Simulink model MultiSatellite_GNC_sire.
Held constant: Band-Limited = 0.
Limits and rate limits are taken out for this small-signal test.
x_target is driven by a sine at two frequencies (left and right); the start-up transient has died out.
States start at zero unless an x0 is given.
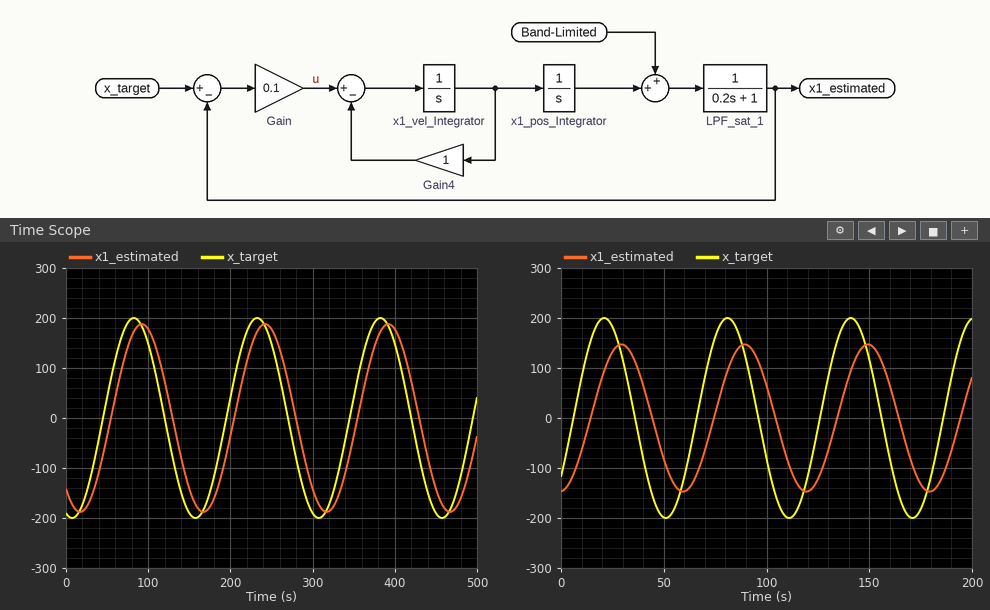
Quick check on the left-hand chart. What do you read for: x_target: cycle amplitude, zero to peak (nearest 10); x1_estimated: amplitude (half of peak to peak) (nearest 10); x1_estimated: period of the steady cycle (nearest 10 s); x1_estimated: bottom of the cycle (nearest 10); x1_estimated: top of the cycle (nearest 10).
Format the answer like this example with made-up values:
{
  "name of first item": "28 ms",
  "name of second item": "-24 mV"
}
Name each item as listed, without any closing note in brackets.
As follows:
{
  "x_target: cycle amplitude, zero to peak": "200",
  "x1_estimated: amplitude (half of peak to peak)": "190",
  "x1_estimated: period of the steady cycle": "150 s",
  "x1_estimated: bottom of the cycle": "-190",
  "x1_estimated: top of the cycle": "190"
}
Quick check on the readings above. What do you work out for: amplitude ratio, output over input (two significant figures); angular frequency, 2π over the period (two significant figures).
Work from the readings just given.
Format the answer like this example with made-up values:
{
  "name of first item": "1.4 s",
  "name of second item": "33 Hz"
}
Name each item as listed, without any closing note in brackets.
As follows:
{
  "amplitude ratio, output over input": "0.95",
  "angular frequency, 2π over the period": "0.042 rad/s"
}
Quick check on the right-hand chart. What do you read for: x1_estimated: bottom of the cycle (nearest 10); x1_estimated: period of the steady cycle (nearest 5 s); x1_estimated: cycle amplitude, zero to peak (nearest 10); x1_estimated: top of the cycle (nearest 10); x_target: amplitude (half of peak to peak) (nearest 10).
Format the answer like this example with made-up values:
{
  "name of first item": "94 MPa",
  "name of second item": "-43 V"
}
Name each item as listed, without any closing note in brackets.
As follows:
{
  "x1_estimated: bottom of the cycle": "-150",
  "x1_estimated: period of the steady cycle": "60 s",
  "x1_estimated: cycle amplitude, zero to peak": "150",
  "x1_estimated: top of the cycle": "150",
  "x_target: amplitude (half of peak to peak)": "200"
}
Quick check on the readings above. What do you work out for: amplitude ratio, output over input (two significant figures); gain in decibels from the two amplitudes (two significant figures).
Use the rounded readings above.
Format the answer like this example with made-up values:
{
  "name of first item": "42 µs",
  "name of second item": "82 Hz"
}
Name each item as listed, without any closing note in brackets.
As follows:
{
  "amplitude ratio, output over input": "0.75",
  "gain in decibels from the two amplitudes": "-2.5 dB"
}
